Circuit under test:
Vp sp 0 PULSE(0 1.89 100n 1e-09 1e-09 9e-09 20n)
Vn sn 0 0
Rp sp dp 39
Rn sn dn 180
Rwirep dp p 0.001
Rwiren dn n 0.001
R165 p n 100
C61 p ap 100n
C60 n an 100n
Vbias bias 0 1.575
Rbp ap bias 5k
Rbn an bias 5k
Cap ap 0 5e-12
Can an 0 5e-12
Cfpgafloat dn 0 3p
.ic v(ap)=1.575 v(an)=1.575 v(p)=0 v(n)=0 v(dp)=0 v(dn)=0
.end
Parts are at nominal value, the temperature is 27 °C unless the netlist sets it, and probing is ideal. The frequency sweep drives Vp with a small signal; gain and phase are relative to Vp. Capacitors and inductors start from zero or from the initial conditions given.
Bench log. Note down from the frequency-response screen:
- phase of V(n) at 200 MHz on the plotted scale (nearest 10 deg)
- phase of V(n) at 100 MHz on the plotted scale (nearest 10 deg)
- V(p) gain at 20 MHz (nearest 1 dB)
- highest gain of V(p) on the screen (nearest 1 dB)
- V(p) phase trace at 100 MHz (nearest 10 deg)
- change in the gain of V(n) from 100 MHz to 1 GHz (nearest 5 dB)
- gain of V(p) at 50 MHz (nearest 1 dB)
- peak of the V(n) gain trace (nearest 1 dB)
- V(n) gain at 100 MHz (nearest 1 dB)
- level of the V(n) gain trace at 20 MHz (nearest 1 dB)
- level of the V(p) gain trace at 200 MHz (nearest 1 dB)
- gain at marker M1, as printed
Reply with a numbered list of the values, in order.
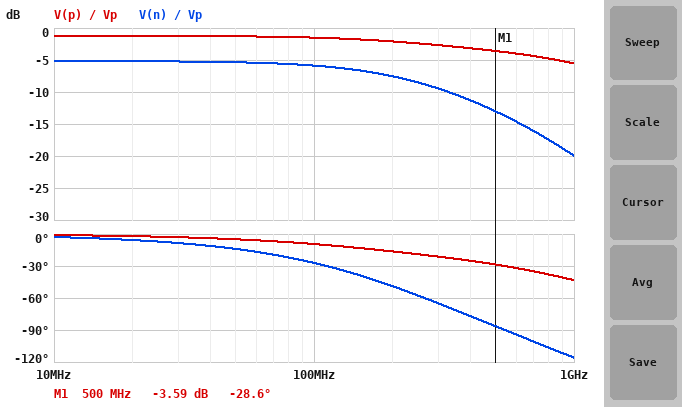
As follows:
1. -50 deg
2. -30 deg
3. -1 dB
4. -1 dB
5. -10 deg
6. -15 dB
7. -1 dB
8. -5 dB
9. -6 dB
10. -5 dB
11. -2 dB
12. -3.59 dB
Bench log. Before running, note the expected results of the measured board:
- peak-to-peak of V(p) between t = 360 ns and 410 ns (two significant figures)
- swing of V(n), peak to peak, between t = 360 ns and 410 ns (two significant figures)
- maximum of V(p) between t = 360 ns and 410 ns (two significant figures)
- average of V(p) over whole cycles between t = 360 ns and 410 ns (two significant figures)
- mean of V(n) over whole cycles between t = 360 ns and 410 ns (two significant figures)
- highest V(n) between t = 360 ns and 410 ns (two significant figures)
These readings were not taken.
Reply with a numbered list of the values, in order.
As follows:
1. 1.6 V
2. 1.0 V
3. 1.6 V
4. 820 mV
5. 520 mV
6. 1.0 V
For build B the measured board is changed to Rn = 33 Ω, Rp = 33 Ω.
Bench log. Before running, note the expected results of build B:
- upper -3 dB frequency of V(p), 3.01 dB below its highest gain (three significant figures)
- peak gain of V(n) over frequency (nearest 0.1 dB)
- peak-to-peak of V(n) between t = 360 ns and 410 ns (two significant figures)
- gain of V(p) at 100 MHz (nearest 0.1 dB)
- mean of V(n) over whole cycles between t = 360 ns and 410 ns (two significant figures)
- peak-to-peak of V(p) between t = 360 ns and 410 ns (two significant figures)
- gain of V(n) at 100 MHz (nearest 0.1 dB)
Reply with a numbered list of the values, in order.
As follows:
1. 1.12 GHz
2. -14.1 dB
3. 370 mV
4. -2.0 dB
5. 190 mV
6. 1.5 V
7. -14.2 dB
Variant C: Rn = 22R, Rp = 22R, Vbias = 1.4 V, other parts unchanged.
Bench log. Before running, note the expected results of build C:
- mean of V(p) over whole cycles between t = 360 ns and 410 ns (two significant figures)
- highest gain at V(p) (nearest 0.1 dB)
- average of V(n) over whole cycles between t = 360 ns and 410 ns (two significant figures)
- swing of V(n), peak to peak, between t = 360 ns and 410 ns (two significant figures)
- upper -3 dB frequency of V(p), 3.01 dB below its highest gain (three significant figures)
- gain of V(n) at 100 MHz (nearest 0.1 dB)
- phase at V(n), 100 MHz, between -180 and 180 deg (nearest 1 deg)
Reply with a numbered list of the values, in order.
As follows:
1. 800 mV
2. -1.5 dB
3. 140 mV
4. 290 mV
5. 1.65 GHz
6. -16.4 dB
7. -9 deg
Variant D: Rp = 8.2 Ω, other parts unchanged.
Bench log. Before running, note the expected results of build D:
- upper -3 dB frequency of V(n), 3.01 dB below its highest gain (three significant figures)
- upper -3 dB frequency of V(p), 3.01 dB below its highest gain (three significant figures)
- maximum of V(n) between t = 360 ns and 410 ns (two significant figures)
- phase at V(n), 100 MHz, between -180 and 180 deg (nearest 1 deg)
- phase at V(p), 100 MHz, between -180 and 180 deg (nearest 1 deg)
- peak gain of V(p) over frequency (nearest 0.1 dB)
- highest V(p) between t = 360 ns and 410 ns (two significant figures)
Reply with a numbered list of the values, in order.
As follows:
1. 296 MHz
2. 3.78 GHz
3. 1.2 V
4. -20 deg
5. -2 deg
6. -0.3 dB
7. 1.8 V
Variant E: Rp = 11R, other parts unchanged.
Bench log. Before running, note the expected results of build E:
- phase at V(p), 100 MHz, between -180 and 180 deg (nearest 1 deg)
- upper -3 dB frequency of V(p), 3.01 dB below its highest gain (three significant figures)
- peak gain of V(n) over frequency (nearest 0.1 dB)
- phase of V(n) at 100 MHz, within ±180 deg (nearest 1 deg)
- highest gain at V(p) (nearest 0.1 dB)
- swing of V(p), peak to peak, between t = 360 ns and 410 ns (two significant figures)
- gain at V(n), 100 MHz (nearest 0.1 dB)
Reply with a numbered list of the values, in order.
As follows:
1. -3 deg
2. 2.78 GHz
3. -4.3 dB
4. -21 deg
5. -0.4 dB
6. 1.8 V
7. -4.8 dB
